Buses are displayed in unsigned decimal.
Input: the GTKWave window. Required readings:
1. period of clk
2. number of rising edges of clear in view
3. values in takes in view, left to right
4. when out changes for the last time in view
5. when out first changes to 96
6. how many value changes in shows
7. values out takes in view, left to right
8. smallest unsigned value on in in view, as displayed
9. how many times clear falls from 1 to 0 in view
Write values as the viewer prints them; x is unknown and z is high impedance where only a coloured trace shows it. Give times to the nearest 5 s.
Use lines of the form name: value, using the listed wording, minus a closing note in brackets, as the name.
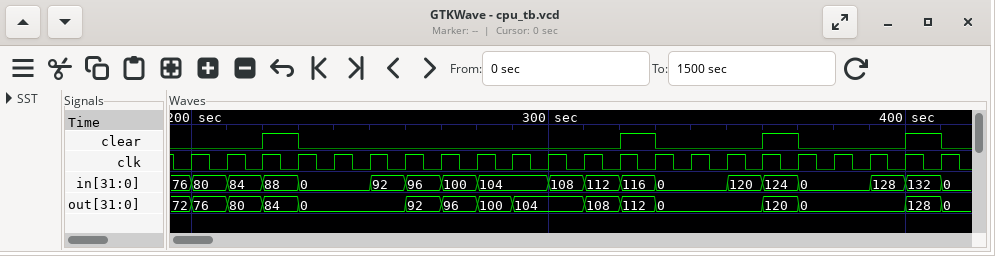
period of clk: 10 s
number of rising edges of clear in view: 4
values in takes in view, left to right: 76, 80, 84, 88, 0, 92, 96, 100, 104, 108, 112, 116, 0, 120, 124, 0, 128, 132, 0
when out changes for the last time in view: 410 s
when out first changes to 96: 270 s
how many value changes in shows: 18
values out takes in view, left to right: 72, 76, 80, 84, 0, 92, 96, 100, 104, 108, 112, 0, 120, 0, 128, 0
smallest unsigned value on in in view, as displayed: 0
how many times clear falls from 1 to 0 in view: 4
